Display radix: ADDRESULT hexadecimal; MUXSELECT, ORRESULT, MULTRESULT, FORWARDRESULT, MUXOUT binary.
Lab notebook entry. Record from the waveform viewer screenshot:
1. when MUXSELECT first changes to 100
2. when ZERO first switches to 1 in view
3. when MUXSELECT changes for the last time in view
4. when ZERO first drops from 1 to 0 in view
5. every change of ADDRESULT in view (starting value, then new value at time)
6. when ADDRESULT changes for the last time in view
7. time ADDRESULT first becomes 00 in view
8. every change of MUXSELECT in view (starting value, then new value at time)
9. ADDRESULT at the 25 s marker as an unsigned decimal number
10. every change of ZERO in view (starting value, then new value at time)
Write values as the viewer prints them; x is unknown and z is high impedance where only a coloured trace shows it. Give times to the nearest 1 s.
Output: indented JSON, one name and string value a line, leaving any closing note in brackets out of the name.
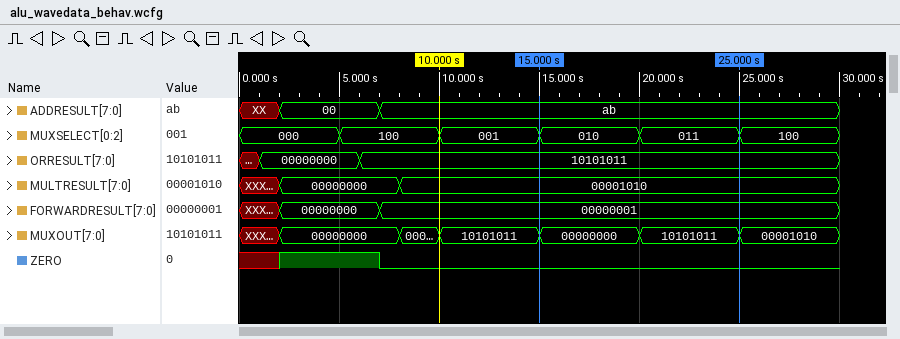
{
  "when MUXSELECT first changes to 100": "5 s",
  "when ZERO first switches to 1 in view": "2 s",
  "when MUXSELECT changes for the last time in view": "25 s",
  "when ZERO first drops from 1 to 0 in view": "7 s",
  "every change of ADDRESULT in view": "XX, 00 at 2 s, ab at 7 s",
  "when ADDRESULT changes for the last time in view": "7 s",
  "time ADDRESULT first becomes 00 in view": "2 s",
  "every change of MUXSELECT in view": "000, 100 at 5 s, 001 at 10 s, 010 at 15 s, 011 at 20 s, 100 at 25 s",
  "ADDRESULT at the 25 s marker as an unsigned decimal number": "171",
  "every change of ZERO in view": "x, 1 at 2 s, 0 at 7 s"
}
